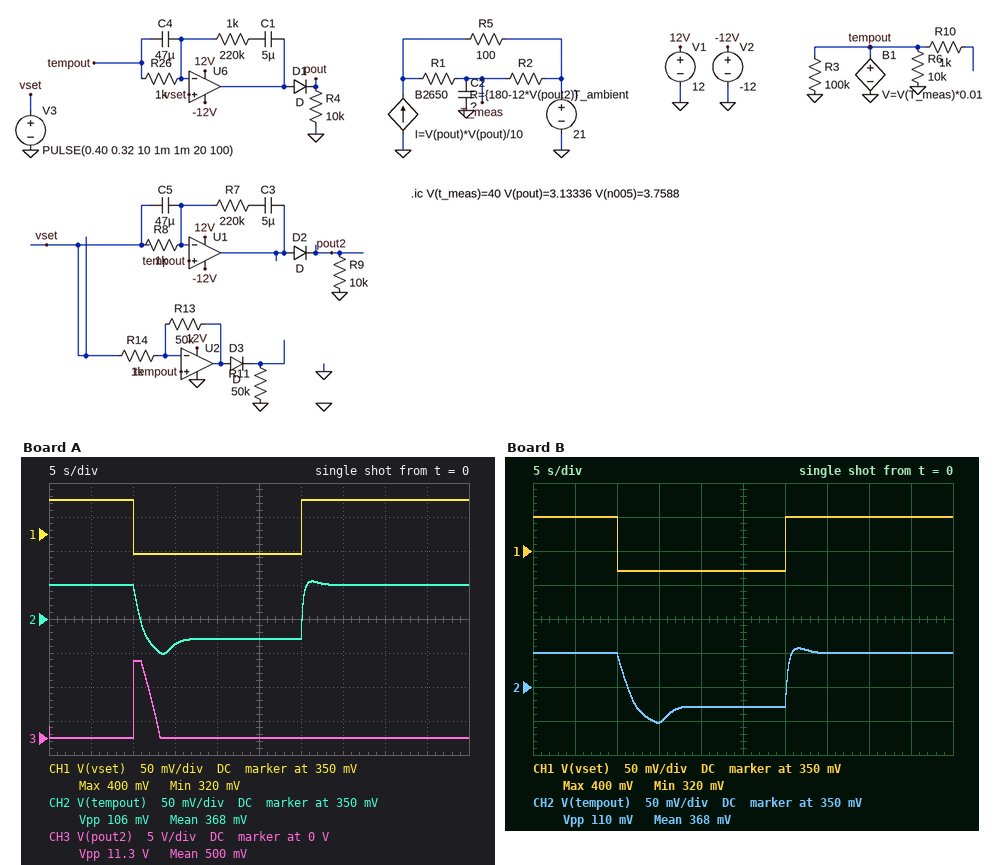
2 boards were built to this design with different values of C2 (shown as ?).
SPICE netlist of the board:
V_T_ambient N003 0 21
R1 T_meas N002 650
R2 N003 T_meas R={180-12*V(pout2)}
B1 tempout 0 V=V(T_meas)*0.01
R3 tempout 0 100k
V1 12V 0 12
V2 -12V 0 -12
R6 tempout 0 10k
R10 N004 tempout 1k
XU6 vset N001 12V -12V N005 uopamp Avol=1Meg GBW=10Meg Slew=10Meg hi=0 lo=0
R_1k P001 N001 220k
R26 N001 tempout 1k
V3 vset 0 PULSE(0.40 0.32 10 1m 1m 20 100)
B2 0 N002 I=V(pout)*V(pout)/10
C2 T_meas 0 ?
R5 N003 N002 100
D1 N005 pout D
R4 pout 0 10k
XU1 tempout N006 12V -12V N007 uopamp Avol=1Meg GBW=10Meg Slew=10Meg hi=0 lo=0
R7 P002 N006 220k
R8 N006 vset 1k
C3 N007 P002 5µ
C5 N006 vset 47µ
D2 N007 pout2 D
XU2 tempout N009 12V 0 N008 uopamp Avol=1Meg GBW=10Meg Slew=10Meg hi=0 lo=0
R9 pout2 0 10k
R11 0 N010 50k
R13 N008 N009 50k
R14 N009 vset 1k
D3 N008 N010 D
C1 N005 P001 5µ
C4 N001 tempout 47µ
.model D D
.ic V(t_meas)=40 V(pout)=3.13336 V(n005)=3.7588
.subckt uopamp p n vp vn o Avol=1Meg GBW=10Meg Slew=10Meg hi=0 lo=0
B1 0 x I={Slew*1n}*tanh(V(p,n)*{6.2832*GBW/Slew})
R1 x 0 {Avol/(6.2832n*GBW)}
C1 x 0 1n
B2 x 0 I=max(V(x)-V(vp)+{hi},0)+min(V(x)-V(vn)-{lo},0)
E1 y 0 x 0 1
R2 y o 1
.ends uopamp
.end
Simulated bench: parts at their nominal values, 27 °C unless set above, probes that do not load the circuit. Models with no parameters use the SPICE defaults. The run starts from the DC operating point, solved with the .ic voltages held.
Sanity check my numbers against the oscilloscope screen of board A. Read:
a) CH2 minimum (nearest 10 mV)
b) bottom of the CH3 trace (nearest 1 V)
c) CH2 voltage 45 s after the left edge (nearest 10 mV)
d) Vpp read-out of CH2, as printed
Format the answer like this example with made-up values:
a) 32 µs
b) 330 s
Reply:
a) 300 mV
b) 0 V
c) 400 mV
d) 106 mV
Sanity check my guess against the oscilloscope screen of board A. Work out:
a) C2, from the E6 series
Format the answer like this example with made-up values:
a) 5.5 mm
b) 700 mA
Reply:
a) 68 mF
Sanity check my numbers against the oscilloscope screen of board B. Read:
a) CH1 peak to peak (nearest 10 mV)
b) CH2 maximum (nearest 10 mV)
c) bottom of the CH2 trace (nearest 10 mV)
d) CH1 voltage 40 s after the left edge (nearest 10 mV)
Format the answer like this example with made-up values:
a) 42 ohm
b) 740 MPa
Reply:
a) 80 mV
b) 410 mV
c) 300 mV
d) 400 mV
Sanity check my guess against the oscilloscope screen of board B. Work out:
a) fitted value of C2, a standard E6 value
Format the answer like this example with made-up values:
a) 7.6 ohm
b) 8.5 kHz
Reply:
a) 100 mF
